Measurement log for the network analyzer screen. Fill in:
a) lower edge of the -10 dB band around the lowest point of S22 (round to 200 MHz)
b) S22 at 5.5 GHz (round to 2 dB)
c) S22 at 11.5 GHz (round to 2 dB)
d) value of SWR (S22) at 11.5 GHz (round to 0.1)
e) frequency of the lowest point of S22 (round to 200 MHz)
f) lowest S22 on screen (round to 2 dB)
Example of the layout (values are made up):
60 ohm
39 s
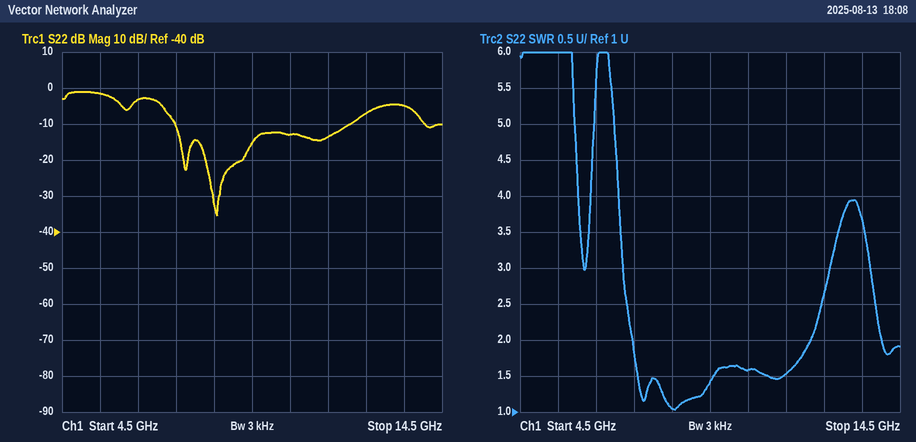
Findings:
7.4 GHz
-2 dB
-14 dB
1.5
8.6 GHz
-36 dB
